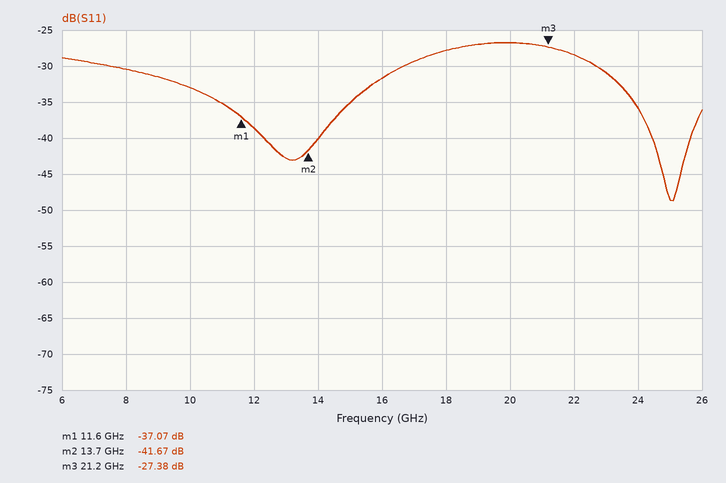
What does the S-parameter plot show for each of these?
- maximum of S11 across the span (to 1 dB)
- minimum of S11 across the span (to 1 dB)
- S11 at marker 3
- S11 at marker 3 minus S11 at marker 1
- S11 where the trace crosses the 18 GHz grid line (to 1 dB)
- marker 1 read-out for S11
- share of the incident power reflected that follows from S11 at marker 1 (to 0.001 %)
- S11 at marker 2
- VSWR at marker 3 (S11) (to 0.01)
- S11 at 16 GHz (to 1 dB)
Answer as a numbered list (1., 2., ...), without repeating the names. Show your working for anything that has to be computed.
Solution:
1. -27 dB
2. -49 dB
3. -27.38 dB
4. -27.38 − (-37.07) = 9.69 dB
5. -28 dB
6. -37.07 dB
7. 10^(-37.07/10) ≈ 0.020 %
8. -41.67 dB
9. (1 + 0.0428)/(1 − 0.0428) ≈ 1.09
10. -32 dB
